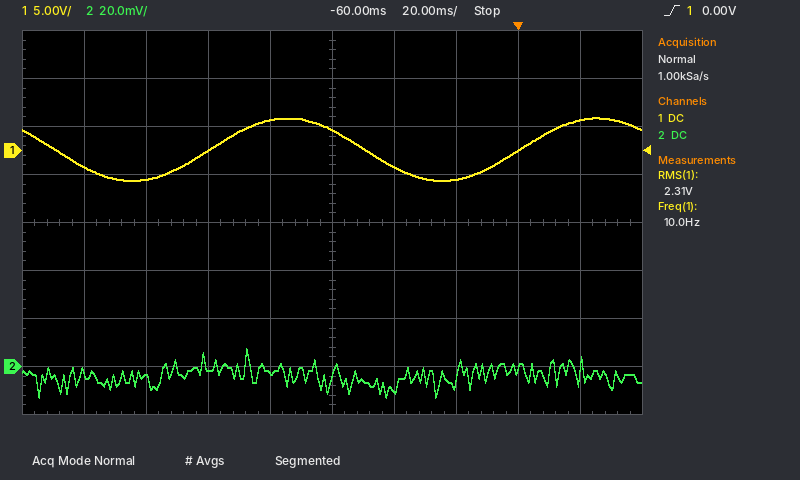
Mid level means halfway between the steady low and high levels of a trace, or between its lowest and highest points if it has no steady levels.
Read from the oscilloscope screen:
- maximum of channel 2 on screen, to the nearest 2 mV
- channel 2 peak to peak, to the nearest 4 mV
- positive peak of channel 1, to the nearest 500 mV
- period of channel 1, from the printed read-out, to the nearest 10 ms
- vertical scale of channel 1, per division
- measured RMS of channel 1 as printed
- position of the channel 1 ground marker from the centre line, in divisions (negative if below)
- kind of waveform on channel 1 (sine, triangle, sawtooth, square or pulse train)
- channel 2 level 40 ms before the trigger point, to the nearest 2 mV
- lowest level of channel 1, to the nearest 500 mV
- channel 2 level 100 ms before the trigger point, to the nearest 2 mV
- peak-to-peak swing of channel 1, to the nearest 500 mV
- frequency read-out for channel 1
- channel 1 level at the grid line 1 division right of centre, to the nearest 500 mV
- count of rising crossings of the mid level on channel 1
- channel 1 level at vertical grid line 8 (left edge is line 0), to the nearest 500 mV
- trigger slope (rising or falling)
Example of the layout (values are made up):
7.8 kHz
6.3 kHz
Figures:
8 mV
20 mV
3.5 V
100 ms
5 V
2.31 V
+1.5 div
sine
-10 mV
-3.0 V
0 mV
6.5 V
10.0 Hz
-1.5 V
2
0.0 V
rising
